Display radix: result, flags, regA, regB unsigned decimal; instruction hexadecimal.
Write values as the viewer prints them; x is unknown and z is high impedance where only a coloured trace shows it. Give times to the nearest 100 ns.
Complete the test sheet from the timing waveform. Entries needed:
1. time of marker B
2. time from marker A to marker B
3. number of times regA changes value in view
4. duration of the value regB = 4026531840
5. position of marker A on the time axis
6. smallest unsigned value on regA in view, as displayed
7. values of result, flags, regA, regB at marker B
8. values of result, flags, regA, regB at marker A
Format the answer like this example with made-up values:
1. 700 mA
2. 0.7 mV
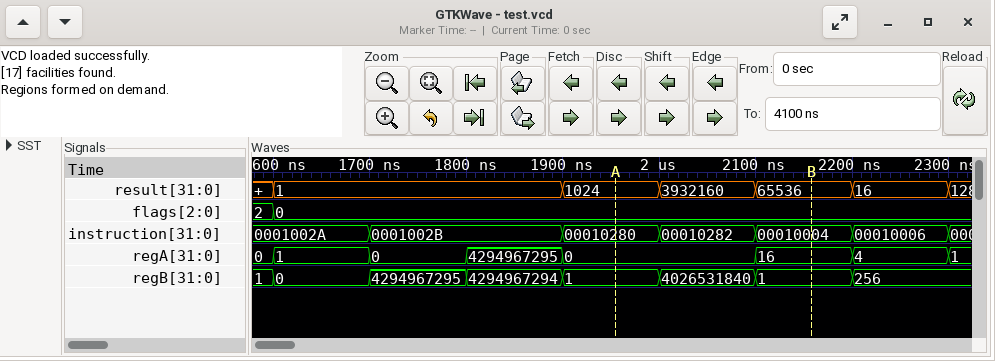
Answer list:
1. 2200 ns
2. 200 ns
3. 7
4. 100 ns
5. 2000 ns
6. 0
7. result=65536, flags=0, regA=16, regB=1
8. result=1024, flags=0, regA=0, regB=1
